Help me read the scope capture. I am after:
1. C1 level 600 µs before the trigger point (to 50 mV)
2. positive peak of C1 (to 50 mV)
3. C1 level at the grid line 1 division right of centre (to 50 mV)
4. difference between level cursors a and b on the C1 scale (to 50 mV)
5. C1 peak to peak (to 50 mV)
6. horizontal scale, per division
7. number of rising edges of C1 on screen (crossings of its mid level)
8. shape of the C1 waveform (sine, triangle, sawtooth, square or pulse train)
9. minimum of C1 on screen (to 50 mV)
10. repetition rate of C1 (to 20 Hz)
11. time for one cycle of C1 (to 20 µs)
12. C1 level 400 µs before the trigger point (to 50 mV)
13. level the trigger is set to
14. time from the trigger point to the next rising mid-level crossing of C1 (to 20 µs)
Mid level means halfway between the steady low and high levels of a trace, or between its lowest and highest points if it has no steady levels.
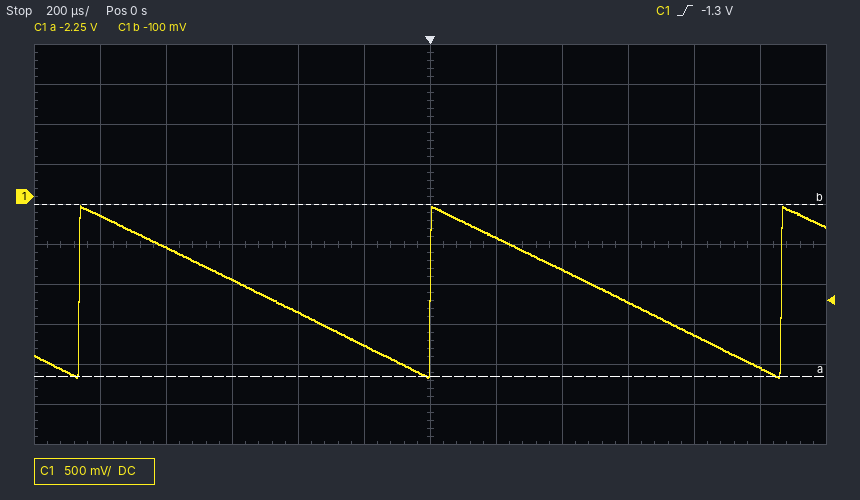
-1.05 V
-100 mV
-500 mV
2.15 V
2.15 V
200 µs
3
sawtooth
-2.25 V
940 Hz
1.06 ms
-1.45 V
-1.3 V
1.06 ms
